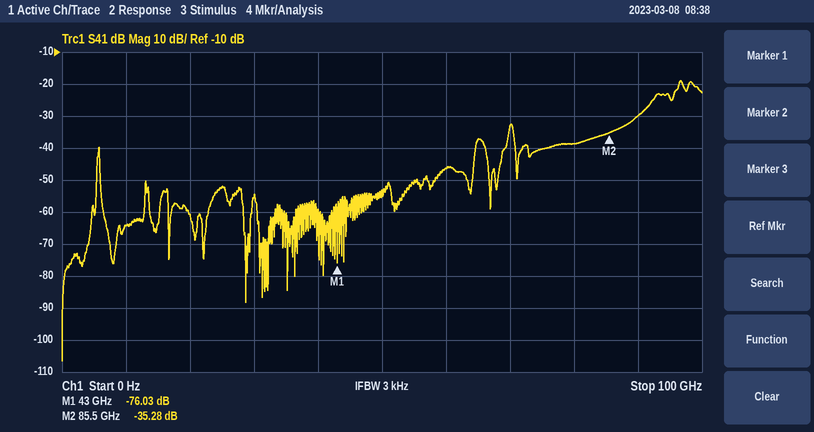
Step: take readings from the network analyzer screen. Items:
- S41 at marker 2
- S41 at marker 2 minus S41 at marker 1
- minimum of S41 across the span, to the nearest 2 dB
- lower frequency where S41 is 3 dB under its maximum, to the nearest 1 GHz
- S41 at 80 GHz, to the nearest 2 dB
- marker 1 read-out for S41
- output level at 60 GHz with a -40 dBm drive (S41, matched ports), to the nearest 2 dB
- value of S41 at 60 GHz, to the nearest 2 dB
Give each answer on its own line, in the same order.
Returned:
-35.28 dB
40.75 dB
-106 dB
96 GHz
-38 dB
-76.03 dB
-86 dBm
-46 dB
